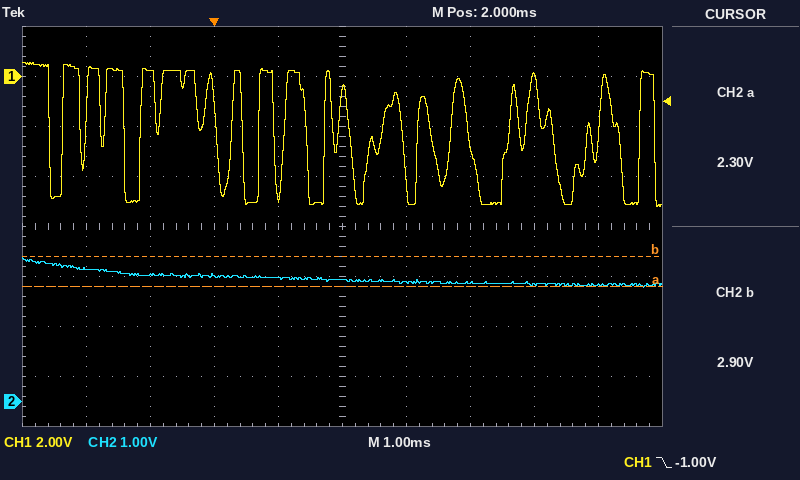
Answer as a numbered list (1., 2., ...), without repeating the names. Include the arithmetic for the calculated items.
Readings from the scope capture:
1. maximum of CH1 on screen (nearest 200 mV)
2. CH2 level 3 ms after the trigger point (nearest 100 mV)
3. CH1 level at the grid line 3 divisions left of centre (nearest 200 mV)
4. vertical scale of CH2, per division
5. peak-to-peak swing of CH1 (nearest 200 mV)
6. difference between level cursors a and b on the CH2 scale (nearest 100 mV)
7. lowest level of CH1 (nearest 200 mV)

1. 600 mV
2. 2.4 V
3. 200 mV
4. 1 V
5. 600 mV − (-5.2 V) = 5.8 V
6. 600 mV
7. -5.2 V
